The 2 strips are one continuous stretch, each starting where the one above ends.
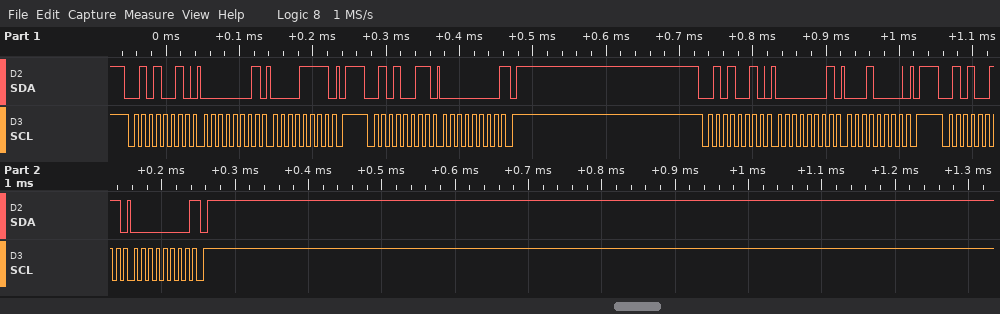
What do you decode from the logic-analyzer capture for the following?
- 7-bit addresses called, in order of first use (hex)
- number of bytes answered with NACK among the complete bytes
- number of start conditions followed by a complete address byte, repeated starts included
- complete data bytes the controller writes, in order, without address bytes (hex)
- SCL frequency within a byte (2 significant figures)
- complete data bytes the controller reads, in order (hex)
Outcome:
0x29
2
4
01 0F 01 10
100 kHz
00 00
